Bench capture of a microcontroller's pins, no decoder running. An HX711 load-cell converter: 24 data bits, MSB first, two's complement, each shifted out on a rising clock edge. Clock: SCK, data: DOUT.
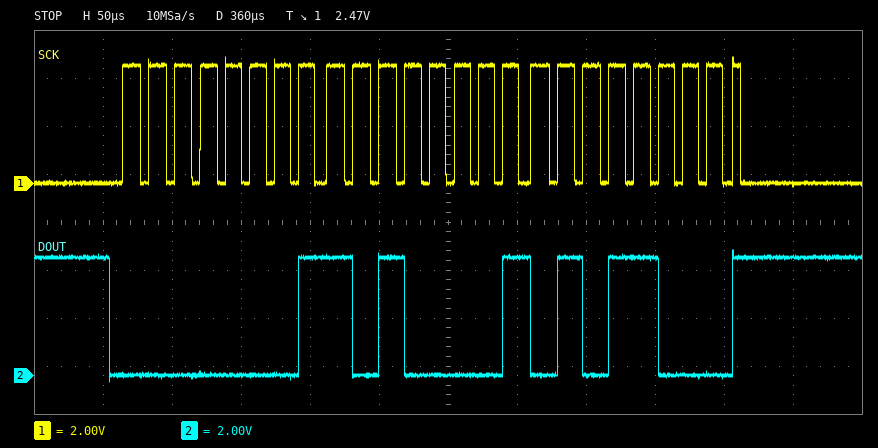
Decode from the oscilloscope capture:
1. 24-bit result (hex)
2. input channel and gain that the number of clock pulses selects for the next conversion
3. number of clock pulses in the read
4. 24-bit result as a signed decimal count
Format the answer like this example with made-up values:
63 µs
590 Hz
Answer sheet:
0x01A158
channel A, gain 128
25
106840
